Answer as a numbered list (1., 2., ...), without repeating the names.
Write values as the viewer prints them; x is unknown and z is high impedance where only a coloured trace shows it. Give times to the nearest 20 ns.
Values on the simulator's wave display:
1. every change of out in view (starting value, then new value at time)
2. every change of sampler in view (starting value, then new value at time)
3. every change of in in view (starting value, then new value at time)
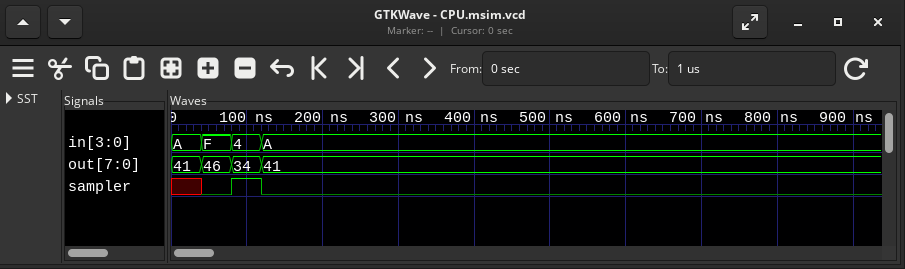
1. 41, 46 at 40 ns, 34 at 80 ns, 41 at 120 ns
2. x, 0 at 40 ns, 1 at 80 ns, 0 at 120 ns
3. A, F at 40 ns, 4 at 80 ns, A at 120 ns
